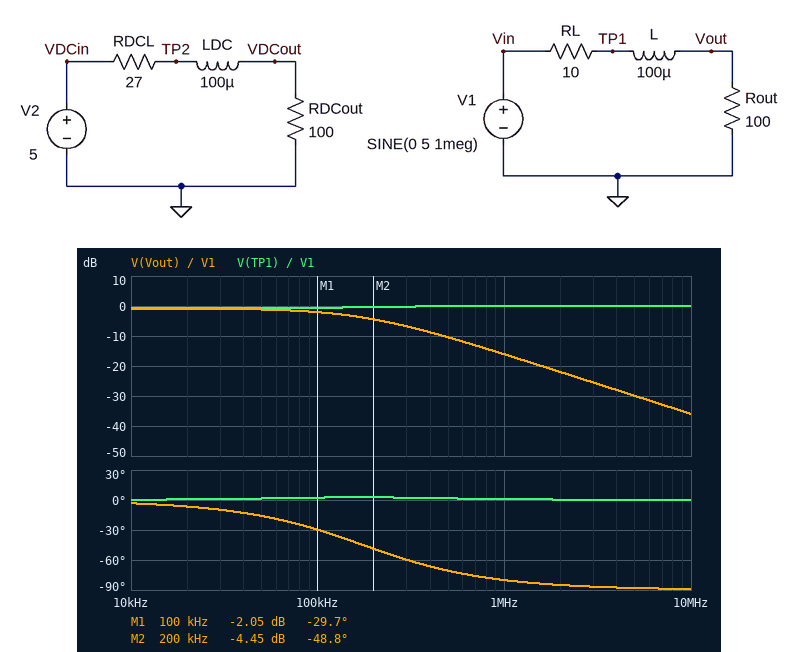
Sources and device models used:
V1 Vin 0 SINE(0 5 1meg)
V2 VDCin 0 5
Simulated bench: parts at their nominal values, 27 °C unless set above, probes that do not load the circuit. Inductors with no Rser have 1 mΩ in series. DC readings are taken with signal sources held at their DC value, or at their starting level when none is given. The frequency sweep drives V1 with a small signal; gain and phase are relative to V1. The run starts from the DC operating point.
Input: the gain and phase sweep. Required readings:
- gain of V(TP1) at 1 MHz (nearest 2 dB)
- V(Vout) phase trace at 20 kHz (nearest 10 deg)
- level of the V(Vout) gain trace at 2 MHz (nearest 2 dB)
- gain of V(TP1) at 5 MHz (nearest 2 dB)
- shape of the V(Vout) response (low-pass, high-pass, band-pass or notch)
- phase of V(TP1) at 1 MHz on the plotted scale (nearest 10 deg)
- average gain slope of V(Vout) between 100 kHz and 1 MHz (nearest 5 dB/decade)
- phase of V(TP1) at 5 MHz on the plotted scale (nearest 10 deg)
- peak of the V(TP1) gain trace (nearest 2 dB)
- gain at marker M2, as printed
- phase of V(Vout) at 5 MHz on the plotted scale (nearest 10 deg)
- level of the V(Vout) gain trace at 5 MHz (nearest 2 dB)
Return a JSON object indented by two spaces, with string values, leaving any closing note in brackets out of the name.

{
  "gain of V(TP1) at 1 MHz": "0 dB",
  "V(Vout) phase trace at 20 kHz": "-10 deg",
  "level of the V(Vout) gain trace at 2 MHz": "-22 dB",
  "gain of V(TP1) at 5 MHz": "0 dB",
  "shape of the V(Vout) response": "low-pass",
  "phase of V(TP1) at 1 MHz on the plotted scale": "0 deg",
  "average gain slope of V(Vout) between 100 kHz and 1 MHz": "-15 dB/decade",
  "phase of V(TP1) at 5 MHz on the plotted scale": "0 deg",
  "peak of the V(TP1) gain trace": "0 dB",
  "gain at marker M2, as printed": "-4.45 dB",
  "phase of V(Vout) at 5 MHz on the plotted scale": "-90 deg",
  "level of the V(Vout) gain trace at 5 MHz": "-30 dB"
}
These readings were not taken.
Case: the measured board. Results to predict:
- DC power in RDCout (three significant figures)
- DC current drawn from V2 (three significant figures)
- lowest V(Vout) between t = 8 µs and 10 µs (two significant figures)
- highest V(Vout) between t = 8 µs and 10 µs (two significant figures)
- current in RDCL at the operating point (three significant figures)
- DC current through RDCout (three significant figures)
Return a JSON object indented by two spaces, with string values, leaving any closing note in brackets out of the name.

{
  "DC power in RDCout": "155 mW",
  "DC current drawn from V2": "39.4 mA",
  "lowest V(Vout) between t = 8 µs and 10 µs": "-780 mV",
  "highest V(Vout) between t = 8 µs and 10 µs": "780 mV",
  "current in RDCL at the operating point": "39.4 mA",
  "DC current through RDCout": "39.4 mA"
}
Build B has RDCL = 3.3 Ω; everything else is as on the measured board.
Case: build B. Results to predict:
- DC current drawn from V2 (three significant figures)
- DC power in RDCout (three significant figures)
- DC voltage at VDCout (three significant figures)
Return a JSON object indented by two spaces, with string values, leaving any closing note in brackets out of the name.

{
  "DC current drawn from V2": "48.4 mA",
  "DC power in RDCout": "234 mW",
  "DC voltage at VDCout": "4.84 V"
}
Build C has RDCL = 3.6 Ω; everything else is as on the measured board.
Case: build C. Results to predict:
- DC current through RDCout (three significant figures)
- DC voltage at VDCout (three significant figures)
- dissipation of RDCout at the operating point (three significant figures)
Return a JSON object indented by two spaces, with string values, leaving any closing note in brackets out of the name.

{
  "DC current through RDCout": "48.3 mA",
  "DC voltage at VDCout": "4.83 V",
  "dissipation of RDCout at the operating point": "233 mW"
}
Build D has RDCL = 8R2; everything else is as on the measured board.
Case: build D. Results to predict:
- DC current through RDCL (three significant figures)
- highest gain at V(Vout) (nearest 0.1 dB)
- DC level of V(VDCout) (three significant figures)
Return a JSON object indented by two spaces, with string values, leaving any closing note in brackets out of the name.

{
  "DC current through RDCL": "46.2 mA",
  "highest gain at V(Vout)": "-0.8 dB",
  "DC level of V(VDCout)": "4.62 V"
}
